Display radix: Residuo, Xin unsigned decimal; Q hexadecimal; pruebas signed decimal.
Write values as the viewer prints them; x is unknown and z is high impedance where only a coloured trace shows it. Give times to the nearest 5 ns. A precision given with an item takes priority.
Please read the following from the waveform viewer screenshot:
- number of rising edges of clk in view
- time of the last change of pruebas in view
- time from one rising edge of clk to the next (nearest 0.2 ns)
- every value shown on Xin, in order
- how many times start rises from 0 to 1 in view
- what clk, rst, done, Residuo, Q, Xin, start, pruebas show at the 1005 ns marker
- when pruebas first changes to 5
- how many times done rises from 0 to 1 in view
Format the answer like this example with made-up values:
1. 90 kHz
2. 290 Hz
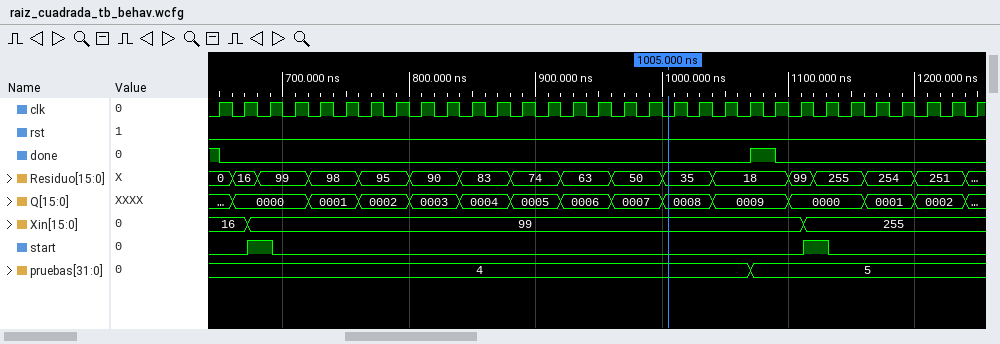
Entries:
1. 31
2. 1070 ns
3. 20 ns
4. 16, 99, 255
5. 2
6. clk=0, rst=0, done=0, Residuo=35, Q=0008, Xin=99, start=0, pruebas=4
7. 1070 ns
8. 1
